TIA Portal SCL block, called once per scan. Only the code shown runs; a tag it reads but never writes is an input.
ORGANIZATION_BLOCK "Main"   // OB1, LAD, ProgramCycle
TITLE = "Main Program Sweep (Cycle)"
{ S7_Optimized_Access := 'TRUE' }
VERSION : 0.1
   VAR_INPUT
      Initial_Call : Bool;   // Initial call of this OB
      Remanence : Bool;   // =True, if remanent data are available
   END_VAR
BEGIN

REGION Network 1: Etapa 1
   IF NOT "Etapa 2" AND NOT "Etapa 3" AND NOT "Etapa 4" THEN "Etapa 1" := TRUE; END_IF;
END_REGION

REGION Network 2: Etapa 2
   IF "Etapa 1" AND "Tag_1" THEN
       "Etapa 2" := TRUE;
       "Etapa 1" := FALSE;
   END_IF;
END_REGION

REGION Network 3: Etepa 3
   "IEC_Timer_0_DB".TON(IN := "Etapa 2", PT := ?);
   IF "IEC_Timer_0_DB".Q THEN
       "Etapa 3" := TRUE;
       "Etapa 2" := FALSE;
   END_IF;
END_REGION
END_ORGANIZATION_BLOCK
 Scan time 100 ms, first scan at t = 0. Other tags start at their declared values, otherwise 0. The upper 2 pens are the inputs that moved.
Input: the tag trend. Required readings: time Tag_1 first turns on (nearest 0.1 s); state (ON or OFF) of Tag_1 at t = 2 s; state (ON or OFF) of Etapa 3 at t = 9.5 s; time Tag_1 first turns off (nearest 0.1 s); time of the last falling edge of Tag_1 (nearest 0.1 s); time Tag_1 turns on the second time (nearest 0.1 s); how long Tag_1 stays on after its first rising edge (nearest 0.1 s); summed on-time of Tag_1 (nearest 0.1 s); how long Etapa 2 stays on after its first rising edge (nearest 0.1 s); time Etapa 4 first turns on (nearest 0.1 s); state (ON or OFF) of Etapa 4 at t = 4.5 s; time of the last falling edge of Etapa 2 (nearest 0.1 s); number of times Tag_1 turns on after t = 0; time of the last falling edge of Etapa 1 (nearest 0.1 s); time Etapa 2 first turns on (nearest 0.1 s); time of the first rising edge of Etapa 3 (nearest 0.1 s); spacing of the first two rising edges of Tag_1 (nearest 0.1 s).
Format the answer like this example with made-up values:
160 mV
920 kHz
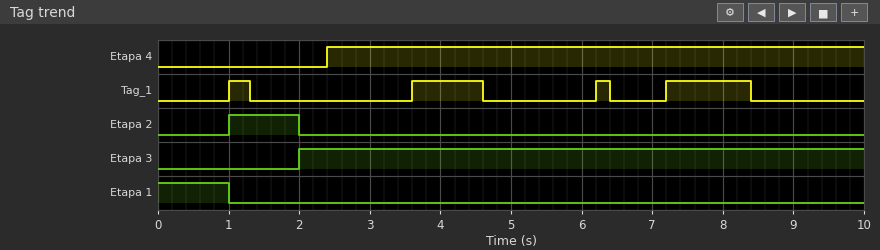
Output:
1.0 s
OFF
ON
1.3 s
8.4 s
3.6 s
0.3 s
2.7 s
1.0 s
2.4 s
ON
2.0 s
4
1.0 s
1.0 s
2.0 s
2.6 s
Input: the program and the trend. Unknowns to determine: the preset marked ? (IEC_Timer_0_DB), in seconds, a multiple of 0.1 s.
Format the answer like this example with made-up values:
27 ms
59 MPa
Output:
1.0 s
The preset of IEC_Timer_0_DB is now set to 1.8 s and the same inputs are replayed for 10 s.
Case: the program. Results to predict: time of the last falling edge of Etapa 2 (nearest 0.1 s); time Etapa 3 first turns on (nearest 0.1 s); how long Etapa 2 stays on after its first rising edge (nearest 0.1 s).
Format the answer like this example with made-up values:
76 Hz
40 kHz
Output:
2.8 s
2.8 s
1.8 s
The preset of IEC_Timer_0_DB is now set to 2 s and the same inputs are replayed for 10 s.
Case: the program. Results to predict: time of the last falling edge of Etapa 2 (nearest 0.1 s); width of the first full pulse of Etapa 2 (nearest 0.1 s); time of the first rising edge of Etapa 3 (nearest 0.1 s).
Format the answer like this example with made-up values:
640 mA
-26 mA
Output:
3.0 s
2.0 s
3.0 s
